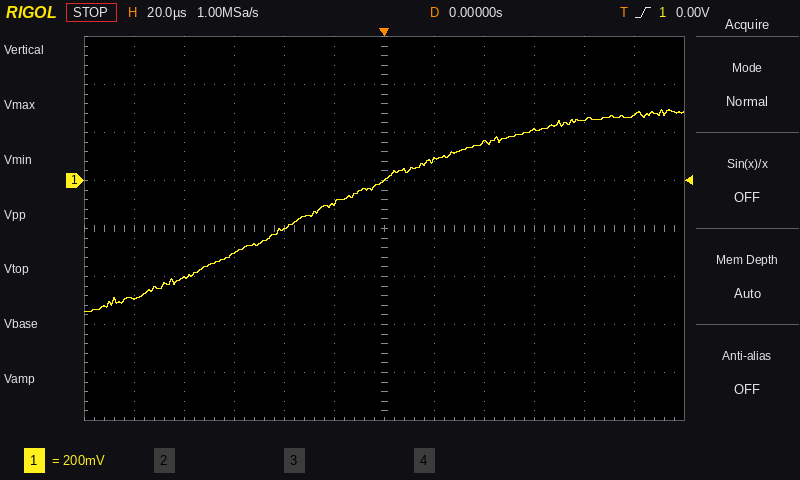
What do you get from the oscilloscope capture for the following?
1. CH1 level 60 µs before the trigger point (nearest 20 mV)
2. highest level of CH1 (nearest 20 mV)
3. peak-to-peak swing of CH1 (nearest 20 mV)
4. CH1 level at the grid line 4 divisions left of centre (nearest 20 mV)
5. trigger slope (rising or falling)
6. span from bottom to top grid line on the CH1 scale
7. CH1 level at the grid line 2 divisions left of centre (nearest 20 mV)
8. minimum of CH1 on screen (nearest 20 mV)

-300 mV
300 mV
840 mV
-400 mV
rising
1.6 V
-200 mV
-540 mV
